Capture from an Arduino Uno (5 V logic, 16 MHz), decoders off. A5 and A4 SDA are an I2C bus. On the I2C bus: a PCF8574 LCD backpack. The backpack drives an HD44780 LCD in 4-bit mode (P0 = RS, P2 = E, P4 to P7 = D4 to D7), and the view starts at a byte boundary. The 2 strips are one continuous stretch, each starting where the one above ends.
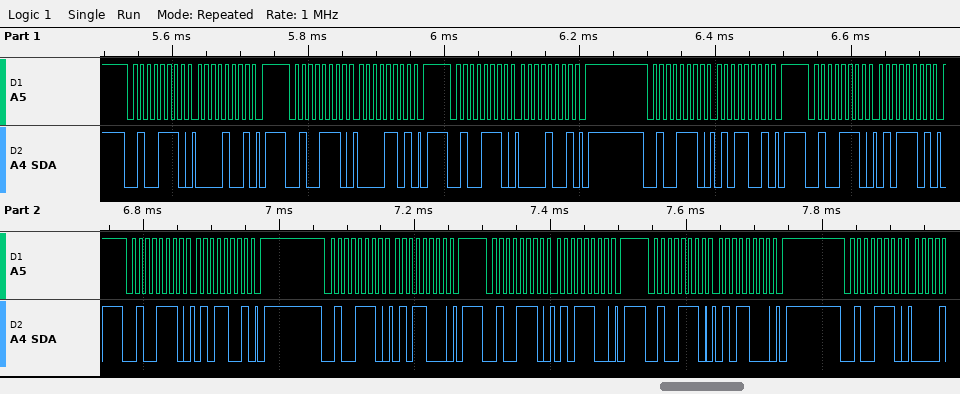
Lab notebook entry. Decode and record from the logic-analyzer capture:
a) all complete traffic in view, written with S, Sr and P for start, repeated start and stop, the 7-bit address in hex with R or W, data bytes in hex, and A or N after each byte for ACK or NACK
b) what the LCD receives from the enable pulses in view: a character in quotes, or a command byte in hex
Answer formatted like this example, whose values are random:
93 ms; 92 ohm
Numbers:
S 27W A 09 A P S 27W A 0D A P S 27W A 09 A P S 27W A 59 A P S 27W A 5D A P S 27W A 59 A P S 27W A 58 A P S 27W A 5C A P S 27W A 58 A P S 27W A; data 0x05
